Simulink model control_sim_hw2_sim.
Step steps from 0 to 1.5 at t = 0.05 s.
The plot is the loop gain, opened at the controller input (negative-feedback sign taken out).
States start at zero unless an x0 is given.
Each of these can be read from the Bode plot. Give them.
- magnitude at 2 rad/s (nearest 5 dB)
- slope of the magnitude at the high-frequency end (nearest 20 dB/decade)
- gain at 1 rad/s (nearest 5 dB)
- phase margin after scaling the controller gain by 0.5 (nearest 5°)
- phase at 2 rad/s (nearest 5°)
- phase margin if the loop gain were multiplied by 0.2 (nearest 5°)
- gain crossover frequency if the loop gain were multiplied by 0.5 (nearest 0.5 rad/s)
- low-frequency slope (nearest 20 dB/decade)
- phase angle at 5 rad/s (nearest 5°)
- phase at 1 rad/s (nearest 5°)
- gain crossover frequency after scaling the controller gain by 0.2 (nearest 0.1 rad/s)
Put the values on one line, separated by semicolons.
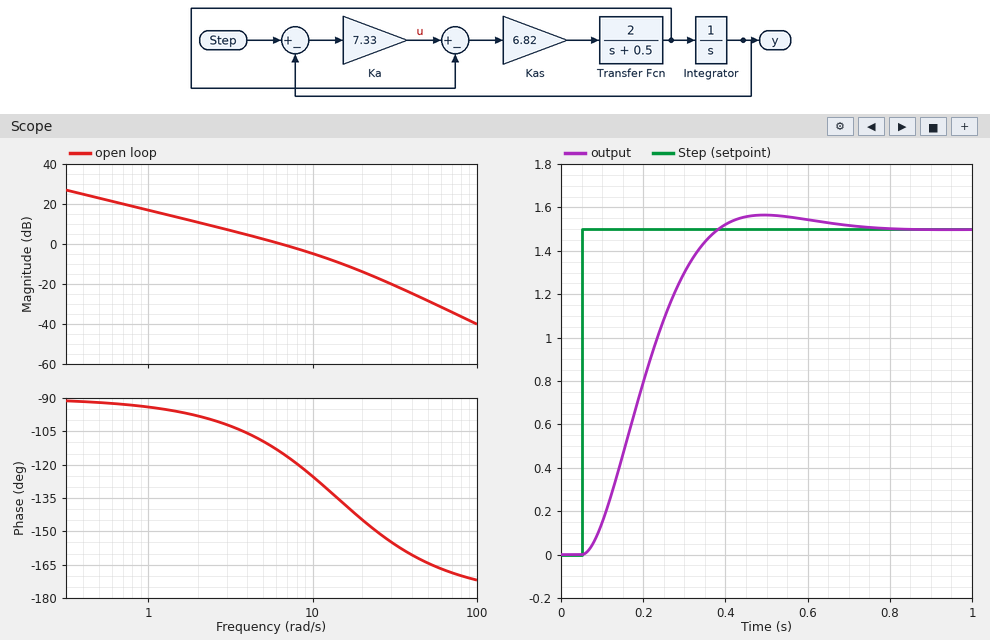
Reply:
10 dB; -40 dB/decade; 15 dB; 75°; -100°; 85°; 3.5 rad/s; -20 dB/decade; -110°; -95°; 1.4 rad/s
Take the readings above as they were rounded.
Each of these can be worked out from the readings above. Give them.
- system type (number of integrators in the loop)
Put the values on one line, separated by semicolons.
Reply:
1
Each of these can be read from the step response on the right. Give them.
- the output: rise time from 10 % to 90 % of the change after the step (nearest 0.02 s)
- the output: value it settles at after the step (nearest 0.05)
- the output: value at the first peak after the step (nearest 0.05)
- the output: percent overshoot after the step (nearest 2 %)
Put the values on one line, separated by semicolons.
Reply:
0.22 s; 1.50; 1.55; 4 %
